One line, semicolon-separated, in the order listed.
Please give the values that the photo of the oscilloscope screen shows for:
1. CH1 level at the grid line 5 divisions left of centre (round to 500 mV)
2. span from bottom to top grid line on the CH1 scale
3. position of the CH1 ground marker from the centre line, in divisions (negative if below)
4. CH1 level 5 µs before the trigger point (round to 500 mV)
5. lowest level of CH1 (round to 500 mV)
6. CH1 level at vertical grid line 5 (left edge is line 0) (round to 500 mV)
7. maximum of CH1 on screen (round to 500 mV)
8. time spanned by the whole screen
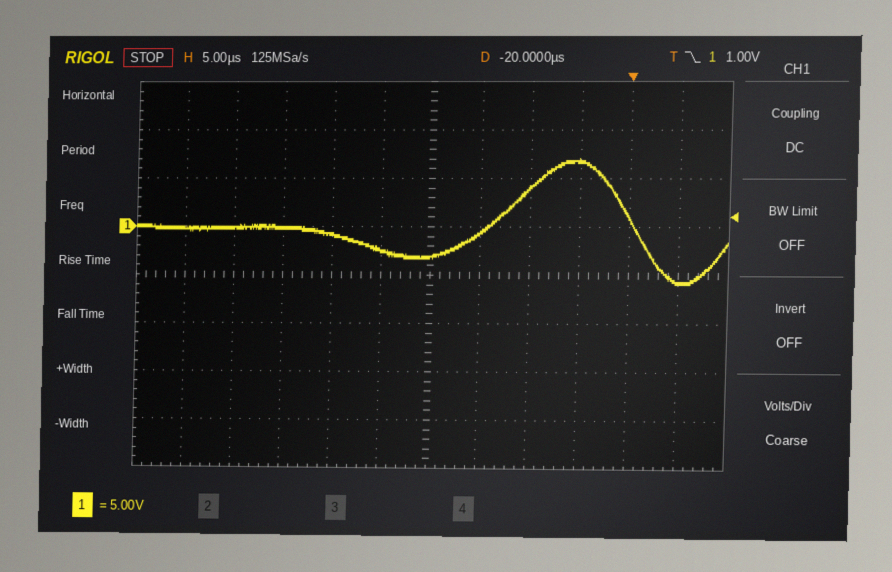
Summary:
0.0 V; 40 V; +1.0 div; 7.0 V; -6.0 V; -2.5 V; 7.0 V; 60 µs
